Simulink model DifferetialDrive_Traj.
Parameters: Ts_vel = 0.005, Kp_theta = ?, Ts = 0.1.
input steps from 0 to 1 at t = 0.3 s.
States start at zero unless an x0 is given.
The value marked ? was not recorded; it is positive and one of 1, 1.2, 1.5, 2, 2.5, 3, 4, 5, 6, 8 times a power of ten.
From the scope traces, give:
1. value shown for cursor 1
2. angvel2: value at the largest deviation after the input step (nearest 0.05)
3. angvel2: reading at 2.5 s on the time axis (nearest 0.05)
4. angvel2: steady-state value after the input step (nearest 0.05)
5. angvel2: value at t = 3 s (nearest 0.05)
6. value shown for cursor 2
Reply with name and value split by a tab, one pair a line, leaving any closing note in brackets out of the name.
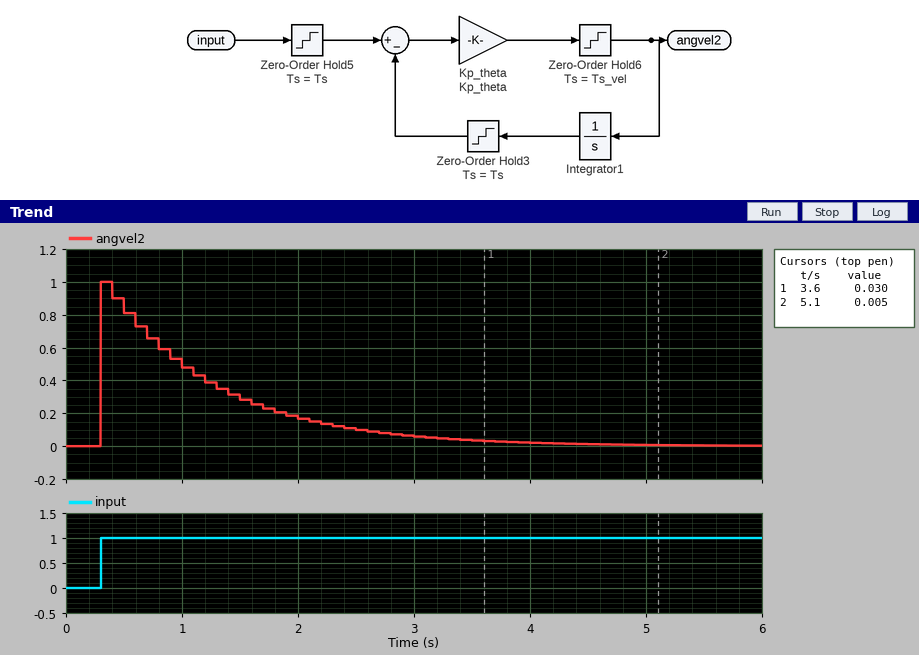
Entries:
value shown for cursor 1	0.030
angvel2: value at the largest deviation after the input step	1.00
angvel2: reading at 2.5 s on the time axis	0.10
angvel2: steady-state value after the input step	0.00
angvel2: value at t = 3 s	0.05
value shown for cursor 2	0.005
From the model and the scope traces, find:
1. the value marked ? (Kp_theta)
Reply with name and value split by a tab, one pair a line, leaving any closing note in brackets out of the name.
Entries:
the value marked ?	1
